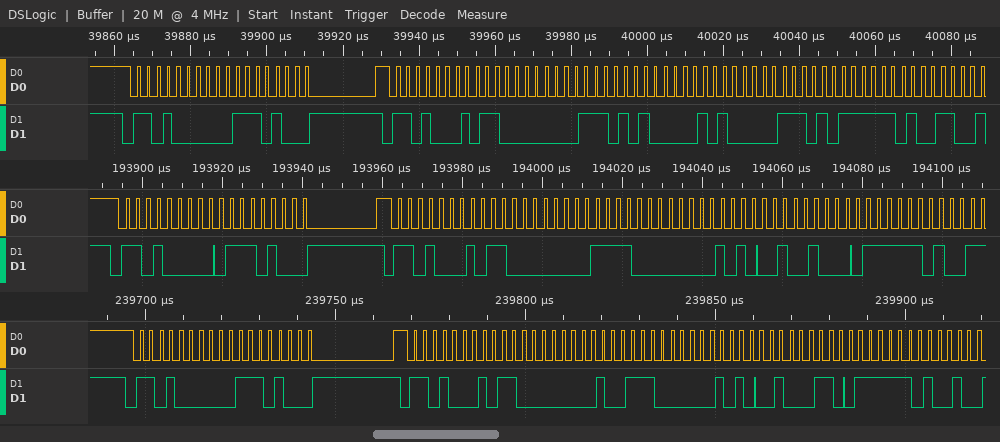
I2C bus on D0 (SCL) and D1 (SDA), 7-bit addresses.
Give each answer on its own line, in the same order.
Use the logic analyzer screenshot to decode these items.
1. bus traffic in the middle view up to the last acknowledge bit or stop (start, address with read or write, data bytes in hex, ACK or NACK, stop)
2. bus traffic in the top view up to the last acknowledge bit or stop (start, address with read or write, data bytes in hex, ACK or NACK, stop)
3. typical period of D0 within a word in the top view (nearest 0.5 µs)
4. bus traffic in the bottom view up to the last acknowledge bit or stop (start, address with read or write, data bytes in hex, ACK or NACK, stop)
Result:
start, address 68 write ACK, 74 ACK, repeated start, address 68 read ACK, C0 ACK, 78 ACK, 0A ACK, 48 ACK, FD ACK
start, address 68 write ACK, 74 ACK, repeated start, address 68 read ACK, C0 ACK, 75 ACK, 0A ACK, 1D ACK, FD ACK
2.5 µs
start, address 68 write ACK, 74 ACK, repeated start, address 68 read ACK, C0 ACK, 4E ACK, 0A ACK, 46 ACK, FD ACK
